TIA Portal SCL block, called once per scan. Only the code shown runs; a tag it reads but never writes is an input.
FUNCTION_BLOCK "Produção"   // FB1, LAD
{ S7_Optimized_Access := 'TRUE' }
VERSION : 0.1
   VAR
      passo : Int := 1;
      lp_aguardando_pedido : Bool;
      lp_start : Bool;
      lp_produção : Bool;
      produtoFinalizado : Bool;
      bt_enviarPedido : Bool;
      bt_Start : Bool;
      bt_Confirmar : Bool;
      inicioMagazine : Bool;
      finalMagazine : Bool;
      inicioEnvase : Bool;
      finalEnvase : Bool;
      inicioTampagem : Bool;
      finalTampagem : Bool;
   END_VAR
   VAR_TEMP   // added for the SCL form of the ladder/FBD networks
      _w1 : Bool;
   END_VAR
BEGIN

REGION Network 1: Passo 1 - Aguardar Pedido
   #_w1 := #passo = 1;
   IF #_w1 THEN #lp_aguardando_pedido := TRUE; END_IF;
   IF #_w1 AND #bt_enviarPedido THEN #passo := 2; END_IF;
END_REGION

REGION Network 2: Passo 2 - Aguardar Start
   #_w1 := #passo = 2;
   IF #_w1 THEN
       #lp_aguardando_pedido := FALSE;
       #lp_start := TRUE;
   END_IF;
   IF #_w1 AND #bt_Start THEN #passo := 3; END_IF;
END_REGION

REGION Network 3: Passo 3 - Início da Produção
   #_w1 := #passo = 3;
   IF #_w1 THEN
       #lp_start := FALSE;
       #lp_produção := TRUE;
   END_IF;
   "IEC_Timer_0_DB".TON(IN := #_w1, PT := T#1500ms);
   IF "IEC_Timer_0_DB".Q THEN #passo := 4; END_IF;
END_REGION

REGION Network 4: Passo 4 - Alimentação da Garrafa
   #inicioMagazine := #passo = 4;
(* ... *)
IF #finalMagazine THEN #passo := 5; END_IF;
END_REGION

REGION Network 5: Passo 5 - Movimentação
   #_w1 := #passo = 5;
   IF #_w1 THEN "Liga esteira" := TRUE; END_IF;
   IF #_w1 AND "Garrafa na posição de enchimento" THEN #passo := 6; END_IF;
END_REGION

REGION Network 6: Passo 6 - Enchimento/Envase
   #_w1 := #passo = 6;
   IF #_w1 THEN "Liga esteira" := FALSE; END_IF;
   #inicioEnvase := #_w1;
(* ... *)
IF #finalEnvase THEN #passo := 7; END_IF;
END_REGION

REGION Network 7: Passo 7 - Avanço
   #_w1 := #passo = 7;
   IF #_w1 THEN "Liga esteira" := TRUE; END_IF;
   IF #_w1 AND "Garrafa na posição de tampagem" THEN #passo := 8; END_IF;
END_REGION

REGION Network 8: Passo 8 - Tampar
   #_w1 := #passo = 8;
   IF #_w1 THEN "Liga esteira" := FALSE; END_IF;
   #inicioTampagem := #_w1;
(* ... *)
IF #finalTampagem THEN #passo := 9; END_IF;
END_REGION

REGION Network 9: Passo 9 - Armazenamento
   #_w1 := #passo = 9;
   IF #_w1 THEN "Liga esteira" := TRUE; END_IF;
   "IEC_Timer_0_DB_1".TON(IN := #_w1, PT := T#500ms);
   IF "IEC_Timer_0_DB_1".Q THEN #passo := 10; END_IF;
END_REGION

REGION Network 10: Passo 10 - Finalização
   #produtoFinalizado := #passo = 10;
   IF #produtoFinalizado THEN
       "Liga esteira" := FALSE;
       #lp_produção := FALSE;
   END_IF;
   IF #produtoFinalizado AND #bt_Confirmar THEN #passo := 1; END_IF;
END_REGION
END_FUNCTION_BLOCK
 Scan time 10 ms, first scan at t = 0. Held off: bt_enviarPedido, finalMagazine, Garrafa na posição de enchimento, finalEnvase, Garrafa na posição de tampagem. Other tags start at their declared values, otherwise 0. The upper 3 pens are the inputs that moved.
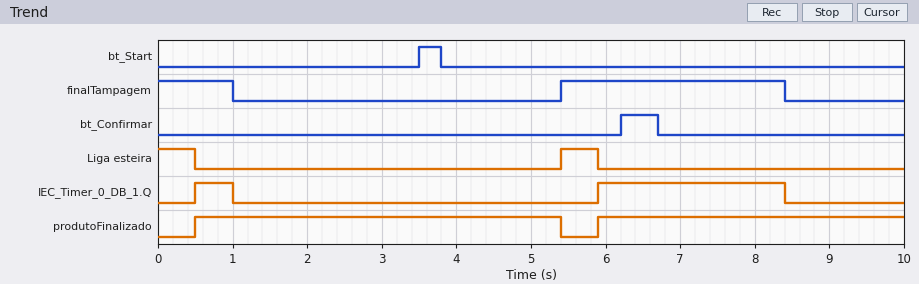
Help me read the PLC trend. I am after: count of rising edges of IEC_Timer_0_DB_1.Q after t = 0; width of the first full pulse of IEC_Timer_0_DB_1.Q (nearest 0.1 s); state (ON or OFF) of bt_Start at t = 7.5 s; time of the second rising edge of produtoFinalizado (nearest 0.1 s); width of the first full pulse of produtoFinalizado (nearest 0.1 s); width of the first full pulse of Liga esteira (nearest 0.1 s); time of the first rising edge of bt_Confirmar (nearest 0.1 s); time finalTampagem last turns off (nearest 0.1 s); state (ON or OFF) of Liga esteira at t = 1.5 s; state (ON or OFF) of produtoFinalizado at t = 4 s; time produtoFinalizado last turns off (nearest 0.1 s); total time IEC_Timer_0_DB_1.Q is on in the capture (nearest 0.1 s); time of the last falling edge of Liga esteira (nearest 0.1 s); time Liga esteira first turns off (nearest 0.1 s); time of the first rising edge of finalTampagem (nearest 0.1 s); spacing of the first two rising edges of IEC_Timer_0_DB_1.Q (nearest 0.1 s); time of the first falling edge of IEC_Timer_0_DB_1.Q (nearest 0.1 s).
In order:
2
0.5 s
OFF
5.9 s
4.9 s
0.5 s
6.2 s
8.4 s
OFF
ON
5.4 s
3.0 s
5.9 s
0.5 s
5.4 s
5.4 s
1.0 s
